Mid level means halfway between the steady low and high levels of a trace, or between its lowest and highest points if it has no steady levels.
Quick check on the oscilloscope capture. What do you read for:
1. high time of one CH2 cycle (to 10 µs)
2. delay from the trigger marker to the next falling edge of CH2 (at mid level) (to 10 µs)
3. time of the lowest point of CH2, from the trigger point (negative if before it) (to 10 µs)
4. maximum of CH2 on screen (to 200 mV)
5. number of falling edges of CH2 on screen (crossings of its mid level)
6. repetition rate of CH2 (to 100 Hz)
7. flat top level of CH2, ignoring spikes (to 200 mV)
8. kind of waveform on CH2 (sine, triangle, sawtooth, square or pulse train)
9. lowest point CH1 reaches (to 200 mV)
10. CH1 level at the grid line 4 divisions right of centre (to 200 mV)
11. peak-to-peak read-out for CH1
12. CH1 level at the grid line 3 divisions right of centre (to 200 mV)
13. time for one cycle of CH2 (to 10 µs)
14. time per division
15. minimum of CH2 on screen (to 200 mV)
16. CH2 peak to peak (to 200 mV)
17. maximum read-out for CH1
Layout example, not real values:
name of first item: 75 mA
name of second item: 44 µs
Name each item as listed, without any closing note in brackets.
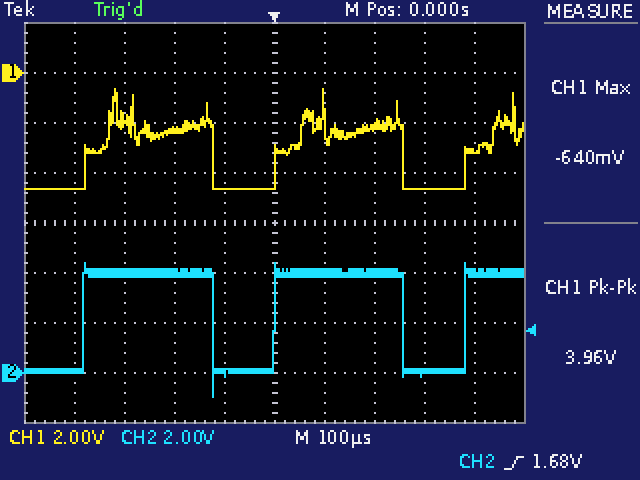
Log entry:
high time of one CH2 cycle: 260 µs
delay from the trigger marker to the next falling edge of CH2 (at mid level): 260 µs
time of the lowest point of CH2, from the trigger point (negative if before it): -120 µs
maximum of CH2 on screen: 4.4 V
number of falling edges of CH2 on screen: 2
repetition rate of CH2: 2.6 kHz
flat top level of CH2, ignoring spikes: 4.0 V
kind of waveform on CH2: pulse train
lowest point CH1 reaches: -4.6 V
CH1 level at the grid line 4 divisions right of centre: -3.2 V
peak-to-peak read-out for CH1: 3.96 V
CH1 level at the grid line 3 divisions right of centre: -4.6 V
time for one cycle of CH2: 380 µs
time per division: 100 µs
minimum of CH2 on screen: -1.0 V
CH2 peak to peak: 5.4 V
maximum read-out for CH1: -640 mV
